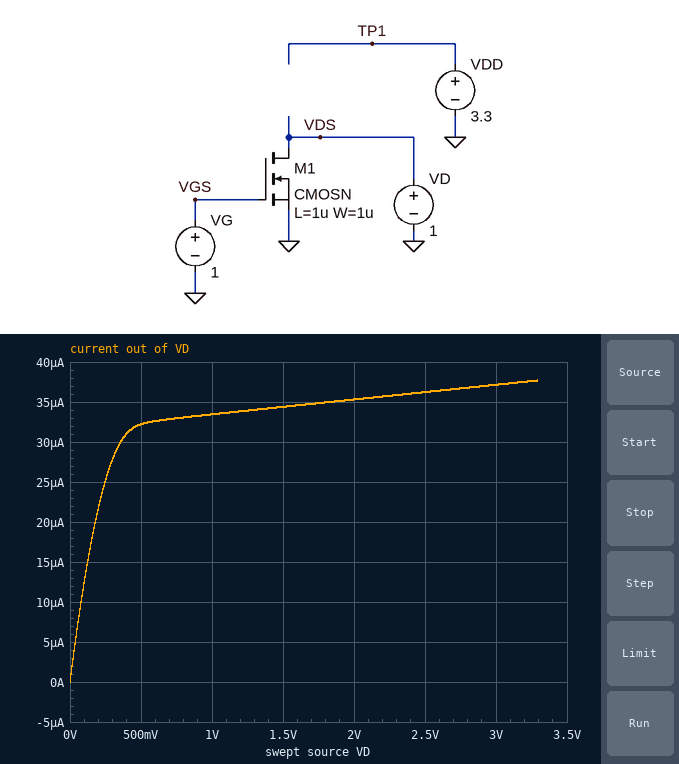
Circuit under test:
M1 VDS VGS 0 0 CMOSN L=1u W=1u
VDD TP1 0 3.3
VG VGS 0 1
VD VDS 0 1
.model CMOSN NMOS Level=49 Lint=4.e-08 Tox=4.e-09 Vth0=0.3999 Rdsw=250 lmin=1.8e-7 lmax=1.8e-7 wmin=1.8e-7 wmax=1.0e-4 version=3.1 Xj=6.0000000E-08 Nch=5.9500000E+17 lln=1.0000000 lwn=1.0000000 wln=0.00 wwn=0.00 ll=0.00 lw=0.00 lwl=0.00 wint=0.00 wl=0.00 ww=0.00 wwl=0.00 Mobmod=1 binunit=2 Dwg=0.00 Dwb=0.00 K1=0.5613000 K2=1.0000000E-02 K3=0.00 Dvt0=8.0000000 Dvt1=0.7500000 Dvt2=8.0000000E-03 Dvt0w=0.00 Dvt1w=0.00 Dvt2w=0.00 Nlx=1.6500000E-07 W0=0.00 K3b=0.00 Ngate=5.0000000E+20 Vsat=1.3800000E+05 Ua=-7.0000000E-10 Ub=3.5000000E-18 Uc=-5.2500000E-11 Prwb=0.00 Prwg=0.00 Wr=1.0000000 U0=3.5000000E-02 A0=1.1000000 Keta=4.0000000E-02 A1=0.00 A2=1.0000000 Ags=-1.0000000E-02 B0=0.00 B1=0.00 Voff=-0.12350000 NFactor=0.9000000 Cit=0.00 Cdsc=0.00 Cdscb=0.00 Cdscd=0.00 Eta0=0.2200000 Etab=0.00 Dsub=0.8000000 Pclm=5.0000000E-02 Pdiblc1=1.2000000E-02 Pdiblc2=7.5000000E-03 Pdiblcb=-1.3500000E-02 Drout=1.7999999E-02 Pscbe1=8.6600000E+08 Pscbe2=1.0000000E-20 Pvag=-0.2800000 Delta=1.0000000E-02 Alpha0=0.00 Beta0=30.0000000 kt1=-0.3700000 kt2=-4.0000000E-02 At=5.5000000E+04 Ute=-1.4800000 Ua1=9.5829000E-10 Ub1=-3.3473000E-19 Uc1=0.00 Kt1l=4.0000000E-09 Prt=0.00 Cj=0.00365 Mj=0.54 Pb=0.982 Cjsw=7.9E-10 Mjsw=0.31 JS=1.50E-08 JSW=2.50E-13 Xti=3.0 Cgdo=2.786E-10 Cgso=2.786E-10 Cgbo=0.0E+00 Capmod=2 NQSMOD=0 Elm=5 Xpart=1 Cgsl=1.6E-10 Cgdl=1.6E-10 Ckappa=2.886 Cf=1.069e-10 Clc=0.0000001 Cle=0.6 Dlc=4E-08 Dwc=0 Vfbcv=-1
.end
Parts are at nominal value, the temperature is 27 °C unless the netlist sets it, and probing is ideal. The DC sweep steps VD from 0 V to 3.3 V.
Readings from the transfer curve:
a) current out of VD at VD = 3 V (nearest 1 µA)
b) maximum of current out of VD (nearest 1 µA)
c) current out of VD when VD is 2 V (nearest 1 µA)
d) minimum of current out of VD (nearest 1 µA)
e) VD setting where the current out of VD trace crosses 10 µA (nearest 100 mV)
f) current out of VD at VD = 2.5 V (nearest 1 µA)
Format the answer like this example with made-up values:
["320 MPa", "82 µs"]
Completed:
["37 µA", "38 µA", "35 µA", "0 A", "100 mV", "36 µA"]
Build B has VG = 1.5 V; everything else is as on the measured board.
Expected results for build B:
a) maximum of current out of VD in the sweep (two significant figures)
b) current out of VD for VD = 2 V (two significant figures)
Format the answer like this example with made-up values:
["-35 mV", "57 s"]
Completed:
["96 µA", "92 µA"]
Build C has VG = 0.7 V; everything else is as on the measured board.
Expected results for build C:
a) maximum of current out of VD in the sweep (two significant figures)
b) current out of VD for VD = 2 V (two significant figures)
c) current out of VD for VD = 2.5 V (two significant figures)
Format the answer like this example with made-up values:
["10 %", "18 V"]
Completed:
["11 µA", "9.9 µA", "10 µA"]
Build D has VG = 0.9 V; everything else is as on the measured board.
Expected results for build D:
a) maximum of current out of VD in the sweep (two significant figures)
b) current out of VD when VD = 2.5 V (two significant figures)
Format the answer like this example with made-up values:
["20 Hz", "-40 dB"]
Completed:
["28 µA", "26 µA"]
